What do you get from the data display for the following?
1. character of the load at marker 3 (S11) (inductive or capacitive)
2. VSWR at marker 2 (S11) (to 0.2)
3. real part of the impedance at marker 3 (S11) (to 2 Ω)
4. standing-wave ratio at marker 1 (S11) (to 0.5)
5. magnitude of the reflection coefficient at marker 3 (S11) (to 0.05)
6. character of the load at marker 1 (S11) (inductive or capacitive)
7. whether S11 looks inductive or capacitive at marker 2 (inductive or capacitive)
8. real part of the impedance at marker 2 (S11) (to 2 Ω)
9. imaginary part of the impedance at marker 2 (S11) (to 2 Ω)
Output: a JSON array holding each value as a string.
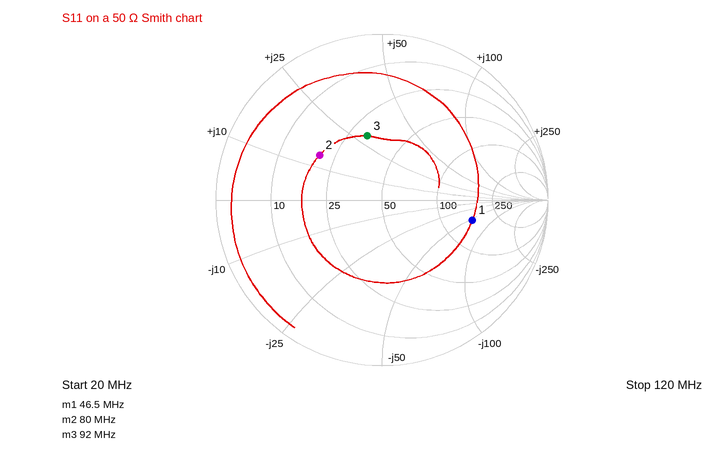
["inductive", "2.8", "32 Ω", "3.5", "0.40", "capacitive", "inductive", "20 Ω", "+14 Ω"]
